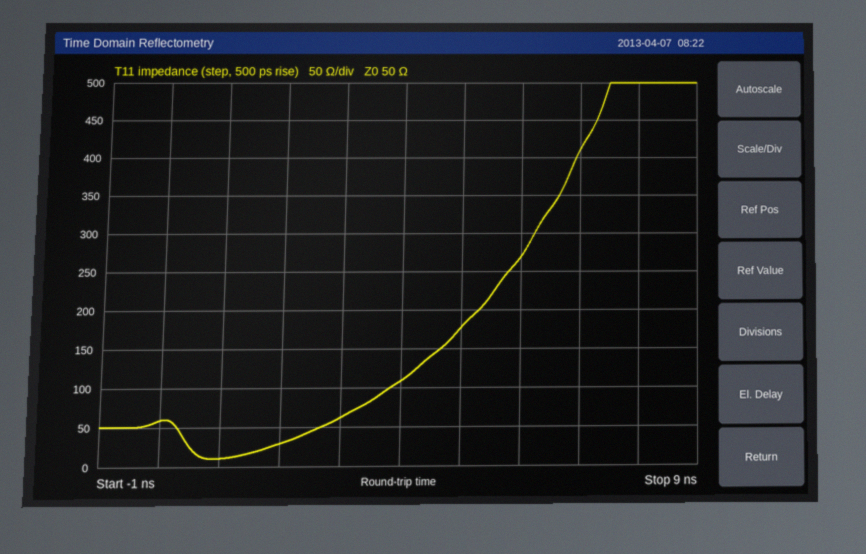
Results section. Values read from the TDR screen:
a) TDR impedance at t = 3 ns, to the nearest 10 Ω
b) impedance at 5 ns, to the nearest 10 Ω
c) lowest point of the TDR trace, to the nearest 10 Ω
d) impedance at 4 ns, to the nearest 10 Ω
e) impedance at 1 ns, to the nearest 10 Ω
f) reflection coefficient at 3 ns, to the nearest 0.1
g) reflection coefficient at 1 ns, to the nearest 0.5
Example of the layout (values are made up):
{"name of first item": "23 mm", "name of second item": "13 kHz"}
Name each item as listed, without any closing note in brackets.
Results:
{"TDR impedance at t = 3 ns, to the nearest 10 Ω": "60 Ω", "impedance at 5 ns, to the nearest 10 Ω": "180 Ω", "lowest point of the TDR trace, to the nearest 10 Ω": "10 Ω", "impedance at 4 ns, to the nearest 10 Ω": "110 Ω", "impedance at 1 ns, to the nearest 10 Ω": "10 Ω", "reflection coefficient at 3 ns, to the nearest 0.1": "+0.1", "reflection coefficient at 1 ns, to the nearest 0.5": "-0.5"}
